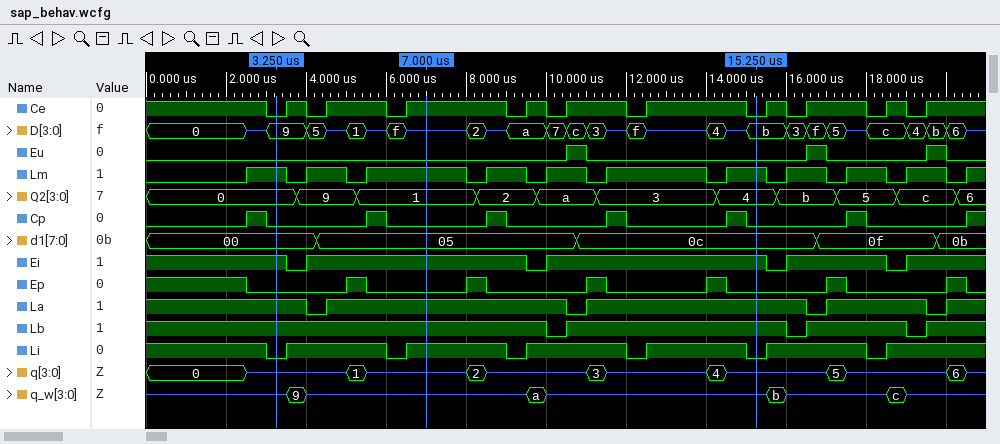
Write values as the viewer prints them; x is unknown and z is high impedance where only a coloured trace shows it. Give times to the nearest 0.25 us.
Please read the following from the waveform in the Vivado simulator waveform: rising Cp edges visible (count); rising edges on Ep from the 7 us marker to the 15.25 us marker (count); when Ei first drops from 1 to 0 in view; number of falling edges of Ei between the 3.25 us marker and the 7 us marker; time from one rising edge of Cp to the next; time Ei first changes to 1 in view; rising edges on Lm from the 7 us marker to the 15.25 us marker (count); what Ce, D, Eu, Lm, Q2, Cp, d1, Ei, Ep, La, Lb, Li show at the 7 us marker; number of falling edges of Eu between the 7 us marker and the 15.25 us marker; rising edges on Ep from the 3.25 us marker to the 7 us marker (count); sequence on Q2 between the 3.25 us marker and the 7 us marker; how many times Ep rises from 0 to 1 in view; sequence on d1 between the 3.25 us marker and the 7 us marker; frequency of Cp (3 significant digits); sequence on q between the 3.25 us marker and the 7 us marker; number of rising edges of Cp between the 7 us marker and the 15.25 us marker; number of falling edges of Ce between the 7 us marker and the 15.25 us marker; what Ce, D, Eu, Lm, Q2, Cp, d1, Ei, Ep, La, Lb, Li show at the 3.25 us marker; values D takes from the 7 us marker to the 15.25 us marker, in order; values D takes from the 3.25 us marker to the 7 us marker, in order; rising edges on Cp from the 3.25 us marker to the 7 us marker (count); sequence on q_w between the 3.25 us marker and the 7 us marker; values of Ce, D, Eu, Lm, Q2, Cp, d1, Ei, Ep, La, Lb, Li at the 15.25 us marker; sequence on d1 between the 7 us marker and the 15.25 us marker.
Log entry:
7
3
3.5 us
1
3 us
4 us
4
Ce=1, D=z, Eu=0, Lm=1, Q2=1, Cp=0, d1=05, Ei=1, Ep=0, La=1, Lb=1, Li=1
1
1
0, 9, 1
6
00, 05
333 kHz
z, 1, z
3
4
Ce=0, D=9, Eu=0, Lm=1, Q2=0, Cp=0, d1=00, Ei=1, Ep=0, La=1, Lb=1, Li=0
z, 2, z, a, 7, c, 3, z, f, z, 4, z, b
9, 5, z, 1, z, f, z
1
z, 9, z
Ce=0, D=b, Eu=0, Lm=1, Q2=4, Cp=0, d1=0c, Ei=1, Ep=0, La=1, Lb=1, Li=0
05, 0c
